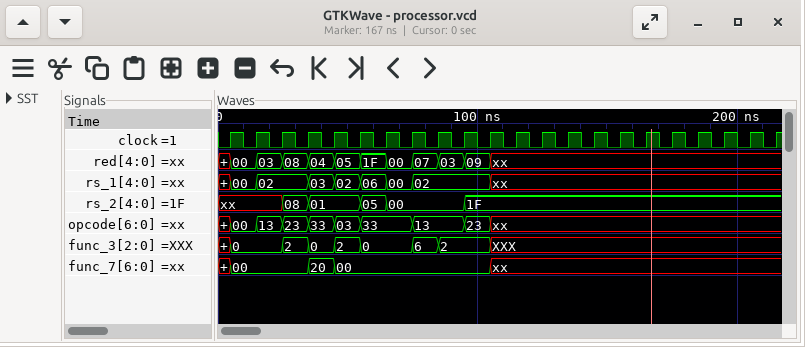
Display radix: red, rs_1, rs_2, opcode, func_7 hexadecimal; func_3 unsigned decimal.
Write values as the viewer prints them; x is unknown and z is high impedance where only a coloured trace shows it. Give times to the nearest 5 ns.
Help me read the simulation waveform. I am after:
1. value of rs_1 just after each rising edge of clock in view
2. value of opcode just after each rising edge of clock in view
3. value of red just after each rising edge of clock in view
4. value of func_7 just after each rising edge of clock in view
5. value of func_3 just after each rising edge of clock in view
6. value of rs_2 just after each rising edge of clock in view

00, 02, 02, 03, 02, 06, 00, 02, 02, 02, xx, xx, xx, xx, xx, xx, xx, xx, xx, xx, xx, xx
00, 13, 23, 33, 03, 33, 33, 13, 13, 23, xx, xx, xx, xx, xx, xx, xx, xx, xx, xx, xx, xx
00, 03, 08, 04, 05, 1F, 00, 07, 03, 09, xx, xx, xx, xx, xx, xx, xx, xx, xx, xx, xx, xx
00, 00, 00, 20, 00, 00, 00, 00, 00, 00, xx, xx, xx, xx, xx, xx, xx, xx, xx, xx, xx, xx
0, 0, 2, 0, 2, 0, 0, 6, 2, 2, XXX, XXX, XXX, XXX, XXX, XXX, XXX, XXX, XXX, XXX, XXX, XXX
xx, xx, 08, 01, 01, 05, 00, 00, 00, 1F, 1F, 1F, 1F, 1F, 1F, 1F, 1F, 1F, 1F, 1F, 1F, 1F
